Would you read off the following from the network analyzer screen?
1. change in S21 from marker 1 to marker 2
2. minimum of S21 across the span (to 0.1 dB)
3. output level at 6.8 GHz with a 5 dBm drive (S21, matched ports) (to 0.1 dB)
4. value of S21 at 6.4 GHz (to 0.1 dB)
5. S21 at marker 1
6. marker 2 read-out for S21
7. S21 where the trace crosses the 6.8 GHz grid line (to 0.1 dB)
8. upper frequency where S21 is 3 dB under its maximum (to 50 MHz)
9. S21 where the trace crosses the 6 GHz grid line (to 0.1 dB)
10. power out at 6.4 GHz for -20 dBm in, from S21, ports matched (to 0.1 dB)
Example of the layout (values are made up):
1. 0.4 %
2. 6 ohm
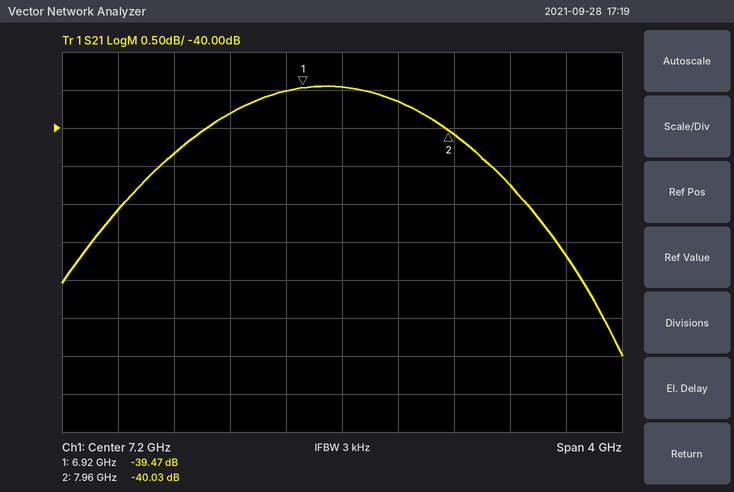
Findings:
1. -0.56 dB
2. -43.0 dB
3. -34.5 dBm
4. -39.8 dB
5. -39.47 dB
6. -40.03 dB
7. -39.5 dB
8. 9.05 GHz
9. -40.3 dB
10. -59.8 dBm
